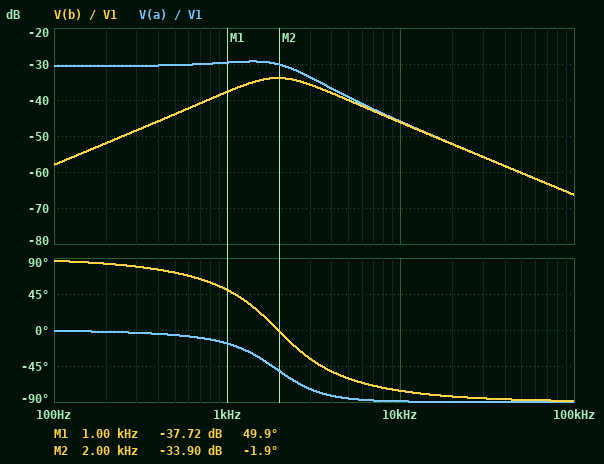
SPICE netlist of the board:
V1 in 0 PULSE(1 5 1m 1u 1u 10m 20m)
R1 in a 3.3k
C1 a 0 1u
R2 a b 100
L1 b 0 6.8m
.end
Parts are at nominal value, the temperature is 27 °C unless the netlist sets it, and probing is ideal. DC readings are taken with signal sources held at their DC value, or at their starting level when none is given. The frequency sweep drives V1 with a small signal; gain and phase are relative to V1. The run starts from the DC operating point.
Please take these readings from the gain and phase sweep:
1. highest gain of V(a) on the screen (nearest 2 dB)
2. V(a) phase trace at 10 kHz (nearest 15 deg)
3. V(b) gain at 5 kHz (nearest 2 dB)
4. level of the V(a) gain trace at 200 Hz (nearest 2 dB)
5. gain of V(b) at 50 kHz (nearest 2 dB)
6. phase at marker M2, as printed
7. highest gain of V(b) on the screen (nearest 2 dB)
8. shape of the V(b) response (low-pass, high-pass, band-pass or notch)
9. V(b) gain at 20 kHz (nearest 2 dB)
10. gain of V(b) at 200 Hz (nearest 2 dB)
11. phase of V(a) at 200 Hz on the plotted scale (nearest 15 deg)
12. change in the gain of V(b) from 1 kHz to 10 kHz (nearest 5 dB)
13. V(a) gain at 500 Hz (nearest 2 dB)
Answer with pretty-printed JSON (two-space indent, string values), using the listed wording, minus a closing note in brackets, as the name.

{
  "highest gain of V(a) on the screen": "-30 dB",
  "V(a) phase trace at 10 kHz": "-90 deg",
  "V(b) gain at 5 kHz": "-40 dB",
  "level of the V(a) gain trace at 200 Hz": "-30 dB",
  "gain of V(b) at 50 kHz": "-60 dB",
  "phase at marker M2, as printed": "-1.9 deg",
  "highest gain of V(b) on the screen": "-34 dB",
  "shape of the V(b) response": "band-pass",
  "V(b) gain at 20 kHz": "-52 dB",
  "gain of V(b) at 200 Hz": "-52 dB",
  "phase of V(a) at 200 Hz on the plotted scale": "0 deg",
  "change in the gain of V(b) from 1 kHz to 10 kHz": "-10 dB",
  "V(a) gain at 500 Hz": "-30 dB"
}
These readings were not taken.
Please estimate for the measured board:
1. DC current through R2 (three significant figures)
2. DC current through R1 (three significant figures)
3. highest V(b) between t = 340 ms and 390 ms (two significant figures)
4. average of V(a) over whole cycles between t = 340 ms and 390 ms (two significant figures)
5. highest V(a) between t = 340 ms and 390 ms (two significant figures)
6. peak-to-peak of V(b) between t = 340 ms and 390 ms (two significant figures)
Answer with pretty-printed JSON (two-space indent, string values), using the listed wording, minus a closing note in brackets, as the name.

{
  "DC current through R2": "294 µA",
  "DC current through R1": "294 µA",
  "highest V(b) between t = 340 ms and 390 ms": "49 mV",
  "average of V(a) over whole cycles between t = 340 ms and 390 ms": "88 mV",
  "highest V(a) between t = 340 ms and 390 ms": "170 mV",
  "peak-to-peak of V(b) between t = 340 ms and 390 ms": "98 mV"
}
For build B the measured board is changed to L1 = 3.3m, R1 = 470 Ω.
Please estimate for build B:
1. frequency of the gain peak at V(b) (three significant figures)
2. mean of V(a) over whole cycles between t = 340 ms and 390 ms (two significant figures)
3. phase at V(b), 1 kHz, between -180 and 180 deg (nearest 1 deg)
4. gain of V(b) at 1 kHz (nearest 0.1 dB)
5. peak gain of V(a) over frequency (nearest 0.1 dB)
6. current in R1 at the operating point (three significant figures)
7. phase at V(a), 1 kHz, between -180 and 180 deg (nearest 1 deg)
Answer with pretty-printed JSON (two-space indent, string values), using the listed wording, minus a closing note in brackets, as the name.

{
  "frequency of the gain peak at V(b)": "3.05 kHz",
  "mean of V(a) over whole cycles between t = 340 ms and 390 ms": "530 mV",
  "phase at V(b), 1 kHz, between -180 and 180 deg": "58 deg",
  "gain of V(b) at 1 kHz": "-29.2 dB",
  "peak gain of V(a) over frequency": "-15.1 dB",
  "current in R1 at the operating point": "1.75 mA",
  "phase at V(a), 1 kHz, between -180 and 180 deg": "-20 deg"
}
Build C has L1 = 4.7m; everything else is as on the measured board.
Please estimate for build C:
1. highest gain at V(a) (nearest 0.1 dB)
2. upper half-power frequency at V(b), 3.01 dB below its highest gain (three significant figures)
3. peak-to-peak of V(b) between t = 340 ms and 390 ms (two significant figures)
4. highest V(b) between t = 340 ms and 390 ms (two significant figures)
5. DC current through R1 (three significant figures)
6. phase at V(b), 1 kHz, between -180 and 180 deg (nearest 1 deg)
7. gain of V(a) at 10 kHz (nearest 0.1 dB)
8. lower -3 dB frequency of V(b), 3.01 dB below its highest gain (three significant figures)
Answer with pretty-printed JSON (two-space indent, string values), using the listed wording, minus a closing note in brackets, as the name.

{
  "highest gain at V(a)": "-30.5 dB",
  "upper half-power frequency at V(b), 3.01 dB below its highest gain": "4.63 kHz",
  "peak-to-peak of V(b) between t = 340 ms and 390 ms": "75 mV",
  "highest V(b) between t = 340 ms and 390 ms": "37 mV",
  "DC current through R1": "294 µA",
  "phase at V(b), 1 kHz, between -180 and 180 deg": "53 deg",
  "gain of V(a) at 10 kHz": "-45.9 dB",
  "lower -3 dB frequency of V(b), 3.01 dB below its highest gain": "1.20 kHz"
}
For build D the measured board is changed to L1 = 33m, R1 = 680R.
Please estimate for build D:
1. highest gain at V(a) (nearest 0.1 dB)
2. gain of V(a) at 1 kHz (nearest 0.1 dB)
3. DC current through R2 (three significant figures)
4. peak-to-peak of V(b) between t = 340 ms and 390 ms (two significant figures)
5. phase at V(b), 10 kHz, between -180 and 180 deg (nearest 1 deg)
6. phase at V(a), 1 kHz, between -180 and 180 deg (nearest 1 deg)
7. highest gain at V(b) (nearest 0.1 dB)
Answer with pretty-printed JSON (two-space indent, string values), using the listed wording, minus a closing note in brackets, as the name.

{
  "highest gain at V(a)": "-8.7 dB",
  "gain of V(a) at 1 kHz": "-8.9 dB",
  "DC current through R2": "1.28 mA",
  "peak-to-peak of V(b) between t = 340 ms and 390 ms": "1.2 V",
  "phase at V(b), 10 kHz, between -180 and 180 deg": "-86 deg",
  "phase at V(a), 1 kHz, between -180 and 180 deg": "-35 deg",
  "highest gain at V(b)": "-9.7 dB"
}
